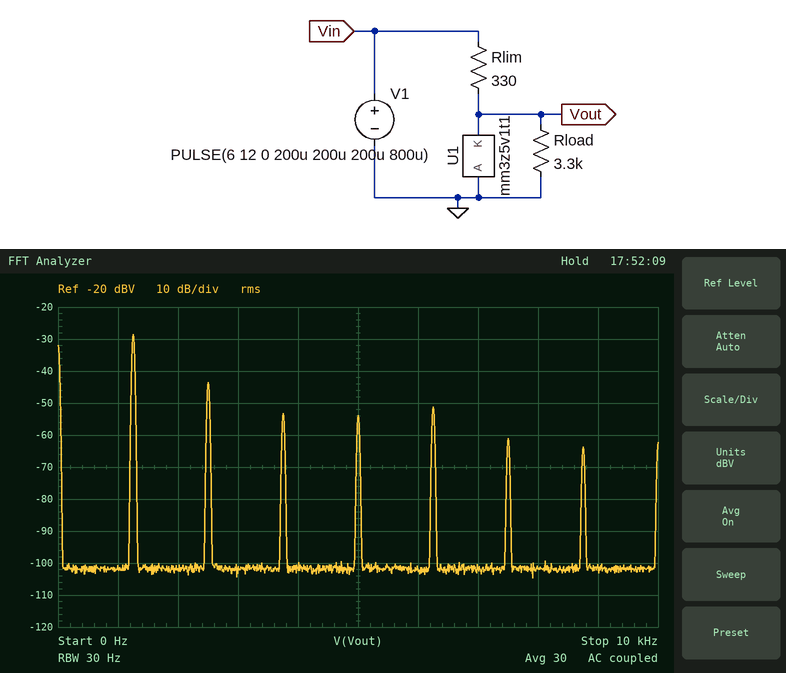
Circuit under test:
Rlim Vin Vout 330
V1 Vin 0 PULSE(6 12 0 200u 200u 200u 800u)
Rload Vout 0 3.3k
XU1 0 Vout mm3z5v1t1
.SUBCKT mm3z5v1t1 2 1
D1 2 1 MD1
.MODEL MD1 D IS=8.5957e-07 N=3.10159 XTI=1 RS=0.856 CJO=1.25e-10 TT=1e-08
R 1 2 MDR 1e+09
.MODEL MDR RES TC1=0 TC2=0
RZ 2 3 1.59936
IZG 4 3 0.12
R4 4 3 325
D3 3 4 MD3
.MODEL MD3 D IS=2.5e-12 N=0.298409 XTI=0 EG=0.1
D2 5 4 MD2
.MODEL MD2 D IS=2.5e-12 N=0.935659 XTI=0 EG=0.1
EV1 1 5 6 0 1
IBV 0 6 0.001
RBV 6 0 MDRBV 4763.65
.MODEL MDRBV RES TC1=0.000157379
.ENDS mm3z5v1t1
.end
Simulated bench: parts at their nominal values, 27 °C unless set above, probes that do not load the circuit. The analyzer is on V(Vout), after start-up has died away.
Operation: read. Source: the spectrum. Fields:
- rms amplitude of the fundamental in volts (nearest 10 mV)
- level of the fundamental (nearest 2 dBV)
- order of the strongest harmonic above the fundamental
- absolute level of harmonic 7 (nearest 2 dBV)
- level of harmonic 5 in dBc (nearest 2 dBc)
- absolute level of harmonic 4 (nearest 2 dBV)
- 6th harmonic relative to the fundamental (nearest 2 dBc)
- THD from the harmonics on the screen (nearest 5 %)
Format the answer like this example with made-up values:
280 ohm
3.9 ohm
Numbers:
40 mV
-28 dBV
2
-64 dBV
-22 dBc
-54 dBV
-32 dBc
20 %
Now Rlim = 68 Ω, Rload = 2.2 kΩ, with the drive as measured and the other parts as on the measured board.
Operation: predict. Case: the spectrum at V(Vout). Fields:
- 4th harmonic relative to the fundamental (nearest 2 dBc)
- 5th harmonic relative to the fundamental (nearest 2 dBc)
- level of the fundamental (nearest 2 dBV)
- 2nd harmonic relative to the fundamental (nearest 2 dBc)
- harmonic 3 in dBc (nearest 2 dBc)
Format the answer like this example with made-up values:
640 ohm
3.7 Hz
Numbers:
-36 dBc
-26 dBc
-22 dBV
-26 dBc
-20 dBc
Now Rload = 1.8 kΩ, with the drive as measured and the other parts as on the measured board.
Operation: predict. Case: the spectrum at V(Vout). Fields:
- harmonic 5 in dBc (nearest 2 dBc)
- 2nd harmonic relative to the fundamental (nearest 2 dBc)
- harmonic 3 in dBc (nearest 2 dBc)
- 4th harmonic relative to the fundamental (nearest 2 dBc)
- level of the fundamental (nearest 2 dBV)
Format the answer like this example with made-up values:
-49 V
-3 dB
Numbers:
-20 dBc
-10 dBc
-42 dBc
-24 dBc
-26 dBV
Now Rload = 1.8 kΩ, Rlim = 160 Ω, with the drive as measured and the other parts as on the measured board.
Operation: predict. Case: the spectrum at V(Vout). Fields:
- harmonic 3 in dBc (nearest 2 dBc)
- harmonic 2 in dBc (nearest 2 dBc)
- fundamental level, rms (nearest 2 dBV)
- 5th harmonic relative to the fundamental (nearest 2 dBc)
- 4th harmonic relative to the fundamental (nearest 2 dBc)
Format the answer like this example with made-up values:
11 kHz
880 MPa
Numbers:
-22 dBc
-18 dBc
-26 dBV
-24 dBc
-28 dBc
